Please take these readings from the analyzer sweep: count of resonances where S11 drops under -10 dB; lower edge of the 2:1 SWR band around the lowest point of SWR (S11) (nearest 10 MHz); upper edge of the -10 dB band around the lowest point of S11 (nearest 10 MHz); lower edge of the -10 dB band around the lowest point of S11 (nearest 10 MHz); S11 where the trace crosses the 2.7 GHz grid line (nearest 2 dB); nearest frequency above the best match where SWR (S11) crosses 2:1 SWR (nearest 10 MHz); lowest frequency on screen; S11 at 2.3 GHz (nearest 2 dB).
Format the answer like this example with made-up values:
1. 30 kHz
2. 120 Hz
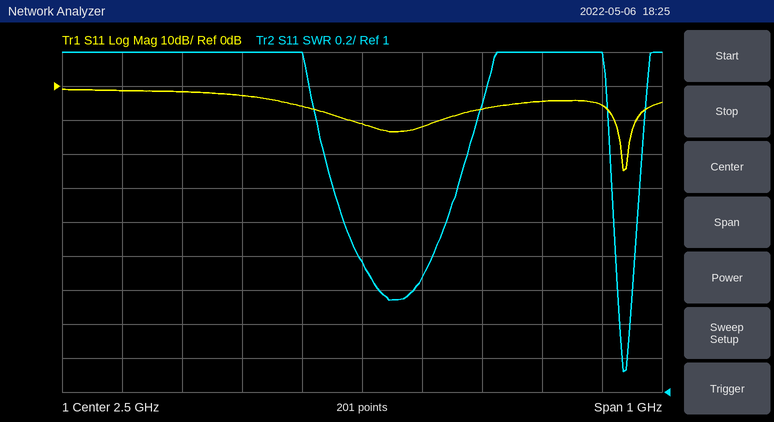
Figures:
1. 2
2. 2.92 GHz
3. 2.96 GHz
4. 2.92 GHz
5. -6 dB
6. 2.96 GHz
7. 2 GHz
8. -2 dB
